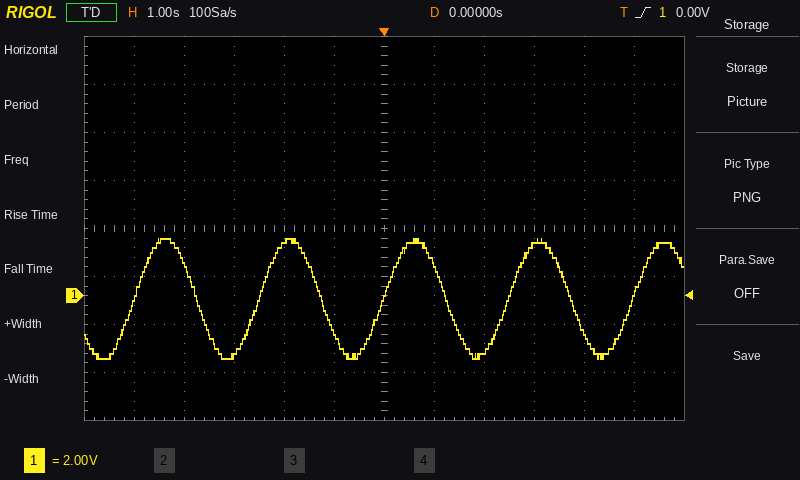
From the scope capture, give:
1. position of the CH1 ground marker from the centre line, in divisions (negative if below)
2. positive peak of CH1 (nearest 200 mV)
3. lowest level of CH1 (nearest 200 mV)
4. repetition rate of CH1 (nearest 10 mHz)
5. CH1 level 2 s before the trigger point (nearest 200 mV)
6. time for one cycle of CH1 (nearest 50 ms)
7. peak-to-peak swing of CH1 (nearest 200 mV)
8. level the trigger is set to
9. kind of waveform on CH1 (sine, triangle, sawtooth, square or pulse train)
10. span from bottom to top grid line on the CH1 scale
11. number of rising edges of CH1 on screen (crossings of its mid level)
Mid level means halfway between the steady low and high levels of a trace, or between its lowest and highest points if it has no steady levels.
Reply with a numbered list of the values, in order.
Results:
1. -1.4 div
2. 2.4 V
3. -2.6 V
4. 400 mHz
5. 2.2 V
6. 2.50 s
7. 5.0 V
8. 0.00 V
9. sine
10. 16 V
11. 5
